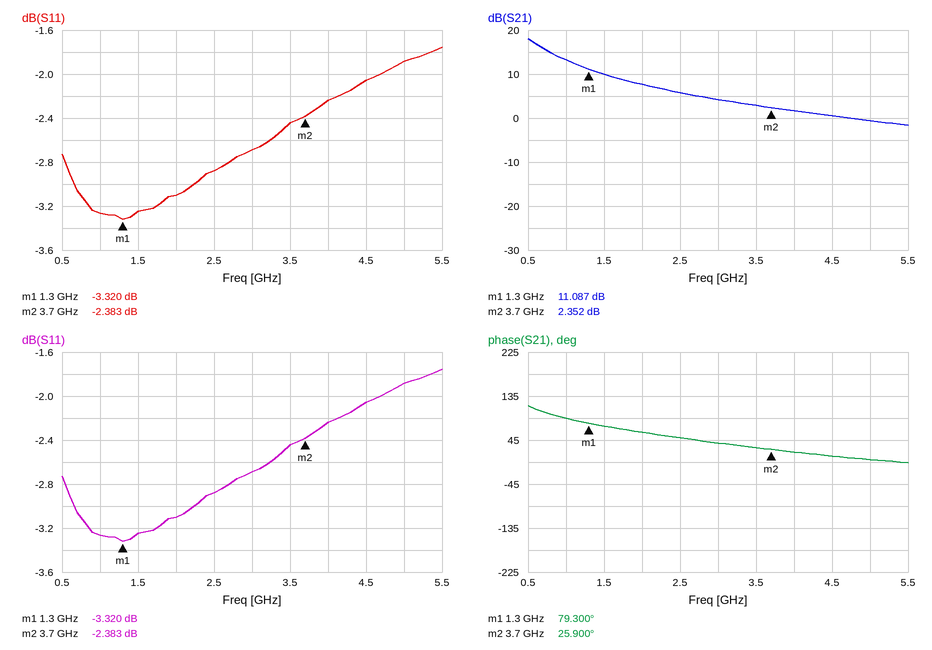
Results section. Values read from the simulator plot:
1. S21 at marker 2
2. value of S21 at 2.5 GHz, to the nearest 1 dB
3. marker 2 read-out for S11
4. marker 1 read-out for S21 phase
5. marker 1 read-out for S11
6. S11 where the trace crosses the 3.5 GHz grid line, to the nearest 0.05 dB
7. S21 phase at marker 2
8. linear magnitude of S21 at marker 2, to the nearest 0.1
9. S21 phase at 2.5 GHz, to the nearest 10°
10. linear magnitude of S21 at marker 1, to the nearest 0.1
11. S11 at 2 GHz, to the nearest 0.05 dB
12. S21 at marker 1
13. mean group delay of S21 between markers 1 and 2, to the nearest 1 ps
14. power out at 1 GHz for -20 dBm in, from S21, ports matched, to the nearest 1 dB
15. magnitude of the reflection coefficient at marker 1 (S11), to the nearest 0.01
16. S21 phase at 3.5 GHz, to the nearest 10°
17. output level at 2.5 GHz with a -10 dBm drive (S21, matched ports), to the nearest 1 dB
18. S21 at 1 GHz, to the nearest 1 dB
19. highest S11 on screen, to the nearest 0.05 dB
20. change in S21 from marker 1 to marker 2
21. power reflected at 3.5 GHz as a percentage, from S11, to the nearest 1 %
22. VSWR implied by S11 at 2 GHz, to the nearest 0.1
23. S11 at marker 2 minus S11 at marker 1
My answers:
2.352 dB
6 dB
-2.383 dB
79.300°
-3.320 dB
-2.45 dB
25.900°
1.3
50°
3.6
-3.10 dB
11.087 dB
62 ps
-7 dBm
0.68
30°
-4 dBm
13 dB
-1.75 dB
-8.735 dB
57 %
5.7
0.937 dB
